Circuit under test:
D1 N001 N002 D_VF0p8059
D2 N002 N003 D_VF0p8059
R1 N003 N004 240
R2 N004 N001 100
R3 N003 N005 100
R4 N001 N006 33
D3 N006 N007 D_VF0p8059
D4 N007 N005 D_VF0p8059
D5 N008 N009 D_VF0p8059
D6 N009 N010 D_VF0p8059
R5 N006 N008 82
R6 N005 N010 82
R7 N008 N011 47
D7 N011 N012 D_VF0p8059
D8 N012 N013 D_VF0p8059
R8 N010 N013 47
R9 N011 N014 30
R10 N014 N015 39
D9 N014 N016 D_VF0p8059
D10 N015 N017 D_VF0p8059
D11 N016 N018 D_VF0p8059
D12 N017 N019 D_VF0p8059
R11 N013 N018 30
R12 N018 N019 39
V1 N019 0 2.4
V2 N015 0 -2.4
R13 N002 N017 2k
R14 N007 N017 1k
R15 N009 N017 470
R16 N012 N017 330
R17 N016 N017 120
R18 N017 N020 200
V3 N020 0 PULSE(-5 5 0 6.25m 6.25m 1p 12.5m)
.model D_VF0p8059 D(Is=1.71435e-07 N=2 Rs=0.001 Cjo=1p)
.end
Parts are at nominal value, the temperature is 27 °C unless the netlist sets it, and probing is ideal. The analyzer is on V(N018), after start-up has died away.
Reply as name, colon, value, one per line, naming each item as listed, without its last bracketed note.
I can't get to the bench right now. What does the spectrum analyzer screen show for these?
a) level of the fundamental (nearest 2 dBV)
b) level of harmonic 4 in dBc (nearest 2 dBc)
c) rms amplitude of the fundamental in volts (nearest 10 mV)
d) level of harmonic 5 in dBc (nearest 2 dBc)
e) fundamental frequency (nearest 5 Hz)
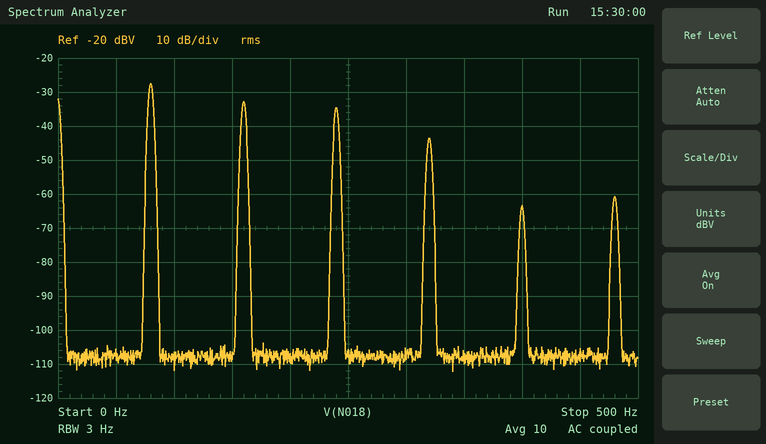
level of the fundamental: -28 dBV
level of harmonic 4 in dBc: -16 dBc
rms amplitude of the fundamental in volts: 40 mV
level of harmonic 5 in dBc: -36 dBc
fundamental frequency: 80 Hz
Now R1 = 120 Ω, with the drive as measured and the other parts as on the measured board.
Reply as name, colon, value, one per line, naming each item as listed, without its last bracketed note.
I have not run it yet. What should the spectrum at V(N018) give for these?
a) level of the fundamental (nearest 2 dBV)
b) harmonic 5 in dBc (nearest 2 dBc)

level of the fundamental: -26 dBV
harmonic 5 in dBc: -32 dBc
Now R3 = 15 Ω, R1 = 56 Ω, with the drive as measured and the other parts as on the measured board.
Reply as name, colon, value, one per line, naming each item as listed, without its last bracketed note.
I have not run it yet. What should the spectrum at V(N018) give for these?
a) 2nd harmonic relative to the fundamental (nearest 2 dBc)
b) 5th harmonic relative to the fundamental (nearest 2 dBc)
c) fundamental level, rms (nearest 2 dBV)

2nd harmonic relative to the fundamental: -8 dBc
5th harmonic relative to the fundamental: -32 dBc
fundamental level, rms: -24 dBV
